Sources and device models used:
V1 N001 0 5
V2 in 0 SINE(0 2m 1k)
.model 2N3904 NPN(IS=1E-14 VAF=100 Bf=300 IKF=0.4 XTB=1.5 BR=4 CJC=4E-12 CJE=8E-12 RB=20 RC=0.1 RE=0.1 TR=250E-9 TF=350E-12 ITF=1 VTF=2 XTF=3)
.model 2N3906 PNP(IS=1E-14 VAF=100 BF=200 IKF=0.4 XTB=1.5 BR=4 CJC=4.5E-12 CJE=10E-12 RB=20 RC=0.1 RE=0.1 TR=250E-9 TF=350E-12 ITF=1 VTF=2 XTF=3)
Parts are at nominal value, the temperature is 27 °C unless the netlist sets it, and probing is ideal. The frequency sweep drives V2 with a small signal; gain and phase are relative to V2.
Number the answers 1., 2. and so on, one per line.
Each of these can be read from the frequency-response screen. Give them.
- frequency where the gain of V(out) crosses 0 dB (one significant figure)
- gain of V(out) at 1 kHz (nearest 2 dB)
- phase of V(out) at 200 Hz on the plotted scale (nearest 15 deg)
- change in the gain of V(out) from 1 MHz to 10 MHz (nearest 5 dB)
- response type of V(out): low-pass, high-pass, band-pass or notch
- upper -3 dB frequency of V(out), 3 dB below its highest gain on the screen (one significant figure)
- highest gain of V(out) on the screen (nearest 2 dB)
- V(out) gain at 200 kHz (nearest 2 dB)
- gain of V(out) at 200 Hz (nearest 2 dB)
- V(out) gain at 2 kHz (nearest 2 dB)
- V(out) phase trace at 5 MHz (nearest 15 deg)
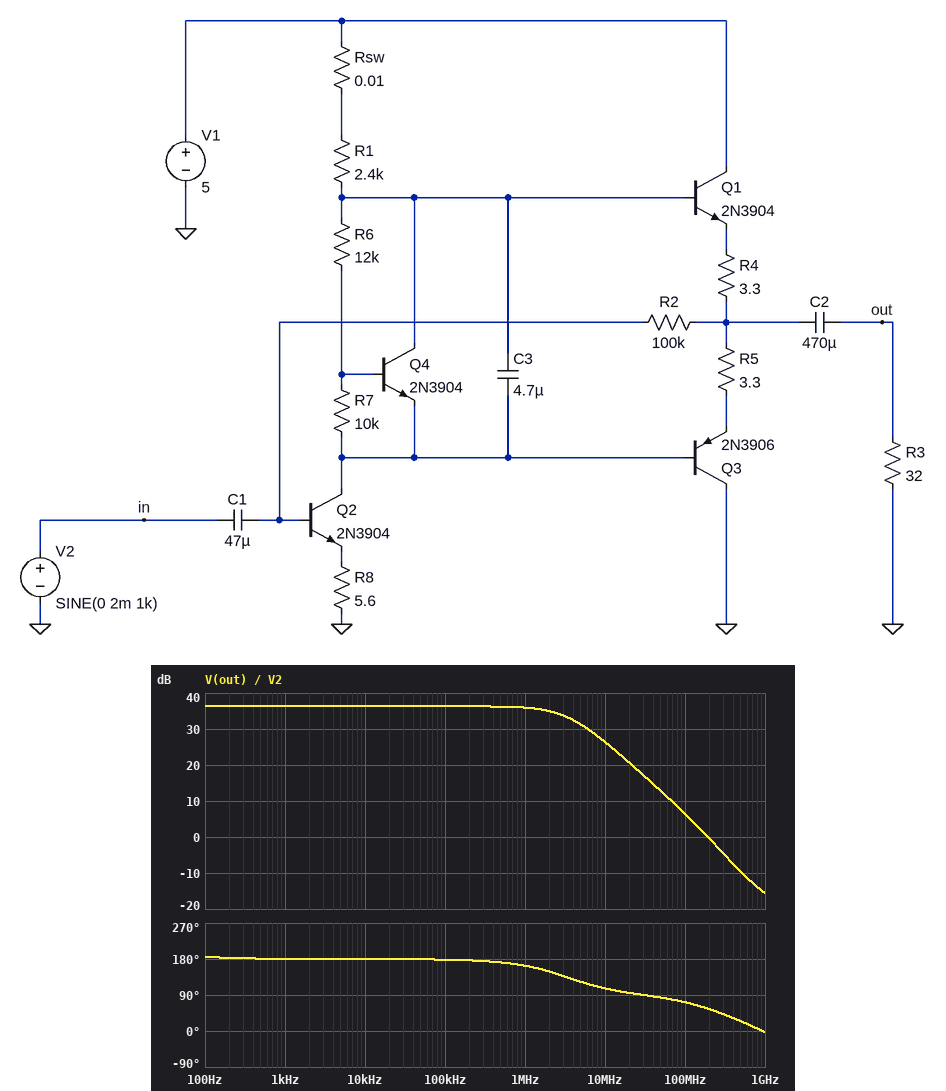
1. 200 MHz
2. 36 dB
3. 180 deg
4. -10 dB
5. low-pass
6. 3 MHz
7. 36 dB
8. 36 dB
9. 36 dB
10. 36 dB
11. 120 deg
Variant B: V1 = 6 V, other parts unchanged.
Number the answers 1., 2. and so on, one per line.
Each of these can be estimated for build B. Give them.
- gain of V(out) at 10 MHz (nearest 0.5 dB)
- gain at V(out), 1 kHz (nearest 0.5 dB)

1. 28.0 dB
2. 38.0 dB
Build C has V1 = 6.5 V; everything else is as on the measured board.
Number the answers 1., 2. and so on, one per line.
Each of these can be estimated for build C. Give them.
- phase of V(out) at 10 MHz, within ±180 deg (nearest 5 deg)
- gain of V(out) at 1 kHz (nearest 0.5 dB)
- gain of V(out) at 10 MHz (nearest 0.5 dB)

1. 105 deg
2. 38.5 dB
3. 29.0 dB
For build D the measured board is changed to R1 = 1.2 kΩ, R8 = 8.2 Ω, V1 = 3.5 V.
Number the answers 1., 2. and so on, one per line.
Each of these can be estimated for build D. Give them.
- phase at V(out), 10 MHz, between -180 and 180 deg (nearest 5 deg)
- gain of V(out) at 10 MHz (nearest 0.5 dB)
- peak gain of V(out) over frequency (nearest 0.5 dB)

1. 120 deg
2. 25.0 dB
3. 31.0 dB
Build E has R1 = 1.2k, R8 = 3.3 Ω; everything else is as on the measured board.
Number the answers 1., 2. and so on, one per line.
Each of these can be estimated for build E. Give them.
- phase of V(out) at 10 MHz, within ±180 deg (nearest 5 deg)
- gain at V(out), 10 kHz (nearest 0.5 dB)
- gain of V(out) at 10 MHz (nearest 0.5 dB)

1. 120 deg
2. 36.0 dB
3. 30.0 dB
